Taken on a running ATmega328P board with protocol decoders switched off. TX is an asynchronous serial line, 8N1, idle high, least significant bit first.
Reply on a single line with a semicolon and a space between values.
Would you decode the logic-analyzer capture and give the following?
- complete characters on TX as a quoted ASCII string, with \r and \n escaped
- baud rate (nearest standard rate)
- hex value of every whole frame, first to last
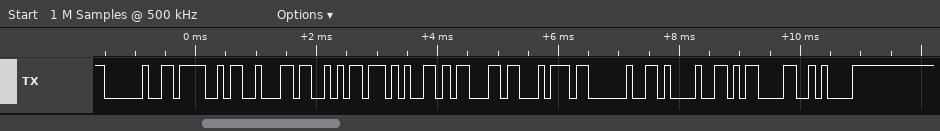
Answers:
" Object !\r\n"; 9600 baud; 0x20 0x4F 0x62 0x6A 0x65 0x63 0x74 0x20 0x21 0x0D 0x0A
